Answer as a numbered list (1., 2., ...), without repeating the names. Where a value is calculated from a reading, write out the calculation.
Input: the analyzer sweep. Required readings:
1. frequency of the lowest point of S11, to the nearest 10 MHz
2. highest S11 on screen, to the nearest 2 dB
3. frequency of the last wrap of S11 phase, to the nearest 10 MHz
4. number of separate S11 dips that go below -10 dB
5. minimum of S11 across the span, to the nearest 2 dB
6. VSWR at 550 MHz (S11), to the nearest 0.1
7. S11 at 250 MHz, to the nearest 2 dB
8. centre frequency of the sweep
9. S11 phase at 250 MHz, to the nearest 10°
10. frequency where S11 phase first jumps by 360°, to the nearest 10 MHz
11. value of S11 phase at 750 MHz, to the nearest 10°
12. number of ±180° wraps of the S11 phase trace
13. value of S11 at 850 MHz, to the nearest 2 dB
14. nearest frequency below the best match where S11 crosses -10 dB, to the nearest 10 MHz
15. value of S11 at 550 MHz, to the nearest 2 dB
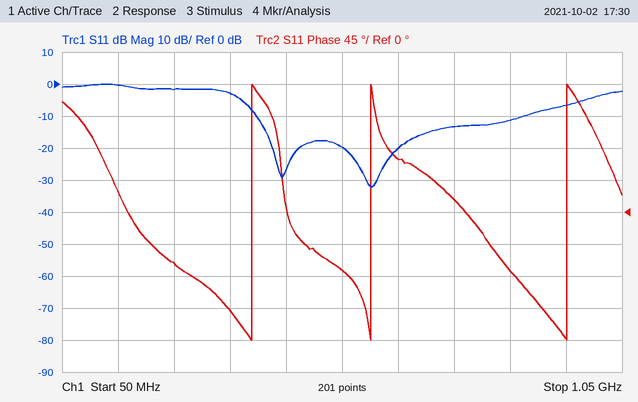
1. 600 MHz
2. 0 dB
3. 950 MHz
4. 2
5. -32 dB
6. |Γ| = 10^(-20/20) = 0.1000; VSWR = (1 + 0.1000)/(1 − 0.1000) ≈ 1.2
7. -2 dB
8. 550 MHz
9. -70°
10. 390 MHz
11. 20°
12. 3
13. -12 dB
14. 400 MHz
15. -20 dB
